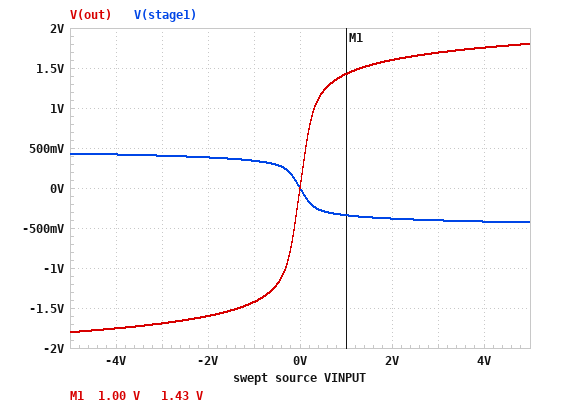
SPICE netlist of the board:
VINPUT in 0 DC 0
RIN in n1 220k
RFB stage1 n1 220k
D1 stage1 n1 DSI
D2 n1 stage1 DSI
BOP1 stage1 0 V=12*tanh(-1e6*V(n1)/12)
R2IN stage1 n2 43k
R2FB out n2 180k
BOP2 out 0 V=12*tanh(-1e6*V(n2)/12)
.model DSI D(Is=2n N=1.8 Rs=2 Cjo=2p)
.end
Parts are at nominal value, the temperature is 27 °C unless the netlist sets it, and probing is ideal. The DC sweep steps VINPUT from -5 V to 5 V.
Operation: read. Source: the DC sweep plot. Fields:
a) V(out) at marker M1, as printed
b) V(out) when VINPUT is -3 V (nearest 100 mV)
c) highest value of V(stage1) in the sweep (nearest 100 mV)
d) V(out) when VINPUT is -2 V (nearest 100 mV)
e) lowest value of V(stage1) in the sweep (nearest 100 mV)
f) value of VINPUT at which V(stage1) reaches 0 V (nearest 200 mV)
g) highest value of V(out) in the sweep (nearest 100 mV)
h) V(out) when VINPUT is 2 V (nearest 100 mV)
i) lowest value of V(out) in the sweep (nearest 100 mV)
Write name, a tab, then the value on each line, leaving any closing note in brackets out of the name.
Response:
V(out) at marker M1, as printed	1.43 V
V(out) when VINPUT is -3 V	-1.7 V
highest value of V(stage1) in the sweep	400 mV
V(out) when VINPUT is -2 V	-1.6 V
lowest value of V(stage1) in the sweep	-400 mV
value of VINPUT at which V(stage1) reaches 0 V	0 V
highest value of V(out) in the sweep	1.8 V
V(out) when VINPUT is 2 V	1.6 V
lowest value of V(out) in the sweep	-1.8 V
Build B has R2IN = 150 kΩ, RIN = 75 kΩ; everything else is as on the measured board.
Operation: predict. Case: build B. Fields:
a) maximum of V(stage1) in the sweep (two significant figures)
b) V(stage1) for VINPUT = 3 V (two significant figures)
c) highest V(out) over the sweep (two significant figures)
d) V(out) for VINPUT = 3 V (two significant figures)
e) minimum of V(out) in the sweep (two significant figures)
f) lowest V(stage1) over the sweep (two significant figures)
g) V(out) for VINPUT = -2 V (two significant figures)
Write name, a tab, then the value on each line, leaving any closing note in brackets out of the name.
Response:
maximum of V(stage1) in the sweep	480 mV
V(stage1) for VINPUT = 3 V	-460 mV
highest V(out) over the sweep	580 mV
V(out) for VINPUT = 3 V	550 mV
minimum of V(out) in the sweep	-580 mV
lowest V(stage1) over the sweep	-480 mV
V(out) for VINPUT = -2 V	-530 mV
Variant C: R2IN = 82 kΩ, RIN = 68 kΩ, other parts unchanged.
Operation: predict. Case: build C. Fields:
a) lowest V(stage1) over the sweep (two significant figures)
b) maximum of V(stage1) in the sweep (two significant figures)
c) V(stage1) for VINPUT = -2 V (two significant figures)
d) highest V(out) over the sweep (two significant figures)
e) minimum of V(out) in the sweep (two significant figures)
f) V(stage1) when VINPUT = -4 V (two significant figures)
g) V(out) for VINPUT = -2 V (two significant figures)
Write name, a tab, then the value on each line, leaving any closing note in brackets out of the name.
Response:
lowest V(stage1) over the sweep	-490 mV
maximum of V(stage1) in the sweep	490 mV
V(stage1) for VINPUT = -2 V	440 mV
highest V(out) over the sweep	1.1 V
minimum of V(out) in the sweep	-1.1 V
V(stage1) when VINPUT = -4 V	480 mV
V(out) for VINPUT = -2 V	-970 mV
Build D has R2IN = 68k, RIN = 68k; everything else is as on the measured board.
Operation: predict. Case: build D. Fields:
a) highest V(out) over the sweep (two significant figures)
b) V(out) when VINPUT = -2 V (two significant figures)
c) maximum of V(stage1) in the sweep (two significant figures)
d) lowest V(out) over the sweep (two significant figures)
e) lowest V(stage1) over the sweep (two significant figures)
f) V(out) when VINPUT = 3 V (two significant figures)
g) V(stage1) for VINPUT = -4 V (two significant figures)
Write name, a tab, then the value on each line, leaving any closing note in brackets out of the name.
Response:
highest V(out) over the sweep	1.3 V
V(out) when VINPUT = -2 V	-1.2 V
maximum of V(stage1) in the sweep	490 mV
lowest V(out) over the sweep	-1.3 V
lowest V(stage1) over the sweep	-490 mV
V(out) when VINPUT = 3 V	1.2 V
V(stage1) for VINPUT = -4 V	480 mV
